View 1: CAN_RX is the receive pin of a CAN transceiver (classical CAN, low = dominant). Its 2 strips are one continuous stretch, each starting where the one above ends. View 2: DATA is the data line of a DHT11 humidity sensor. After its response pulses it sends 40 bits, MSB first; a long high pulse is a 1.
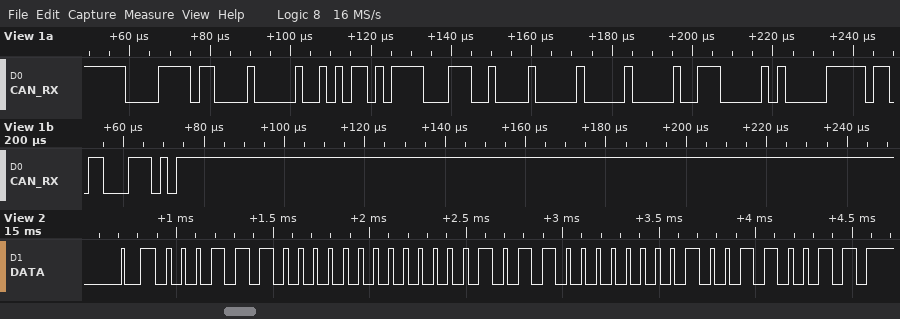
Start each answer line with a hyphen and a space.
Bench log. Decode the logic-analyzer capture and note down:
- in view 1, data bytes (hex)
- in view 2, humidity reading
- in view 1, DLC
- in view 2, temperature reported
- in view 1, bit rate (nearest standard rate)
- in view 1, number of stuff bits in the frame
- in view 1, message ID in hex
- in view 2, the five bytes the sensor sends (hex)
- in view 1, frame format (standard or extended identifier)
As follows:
- 0A D7 8E 42 00 00 E0 41
- 28 %
- 8
- 22.1 °C
- 500 kbit/s
- 7
- 0x0F6
- 1C 00 16 01 33
- standard
